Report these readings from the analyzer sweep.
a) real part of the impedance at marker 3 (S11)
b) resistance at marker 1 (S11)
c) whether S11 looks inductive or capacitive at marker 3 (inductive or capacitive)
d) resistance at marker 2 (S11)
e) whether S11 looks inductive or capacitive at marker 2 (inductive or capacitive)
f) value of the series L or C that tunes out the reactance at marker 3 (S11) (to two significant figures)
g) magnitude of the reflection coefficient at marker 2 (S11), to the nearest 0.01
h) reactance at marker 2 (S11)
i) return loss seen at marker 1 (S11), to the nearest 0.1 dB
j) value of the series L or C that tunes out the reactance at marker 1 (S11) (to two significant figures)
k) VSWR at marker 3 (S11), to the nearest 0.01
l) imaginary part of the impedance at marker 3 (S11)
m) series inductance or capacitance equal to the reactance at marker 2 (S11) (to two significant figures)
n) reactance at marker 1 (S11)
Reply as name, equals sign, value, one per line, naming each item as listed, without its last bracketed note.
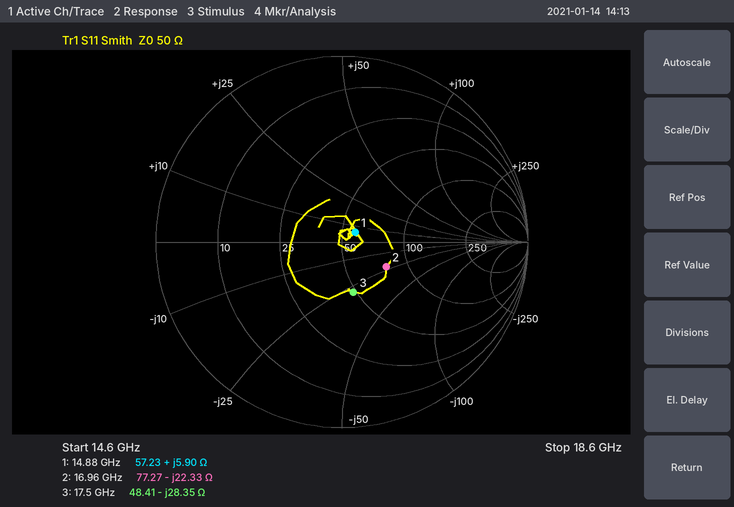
real part of the impedance at marker 3 = 48.41 Ω
resistance at marker 1 = 57.23 Ω
whether S11 looks inductive or capacitive at marker 3 = capacitive
resistance at marker 2 = 77.27 Ω
whether S11 looks inductive or capacitive at marker 2 = capacitive
value of the series L or C that tunes out the reactance at marker 3 (S11) = 260 pH
magnitude of the reflection coefficient at marker 2 (S11), to the nearest 0.01 = 0.27
reactance at marker 2 = -22.33 Ω
return loss seen at marker 1 (S11), to the nearest 0.1 dB = 21.2 dB
value of the series L or C that tunes out the reactance at marker 1 (S11) = 1.8 pF
VSWR at marker 3 (S11), to the nearest 0.01 = 1.77
imaginary part of the impedance at marker 3 = -28.35 Ω
series inductance or capacitance equal to the reactance at marker 2 (S11) = 420 fF
reactance at marker 1 = +5.90 Ω
